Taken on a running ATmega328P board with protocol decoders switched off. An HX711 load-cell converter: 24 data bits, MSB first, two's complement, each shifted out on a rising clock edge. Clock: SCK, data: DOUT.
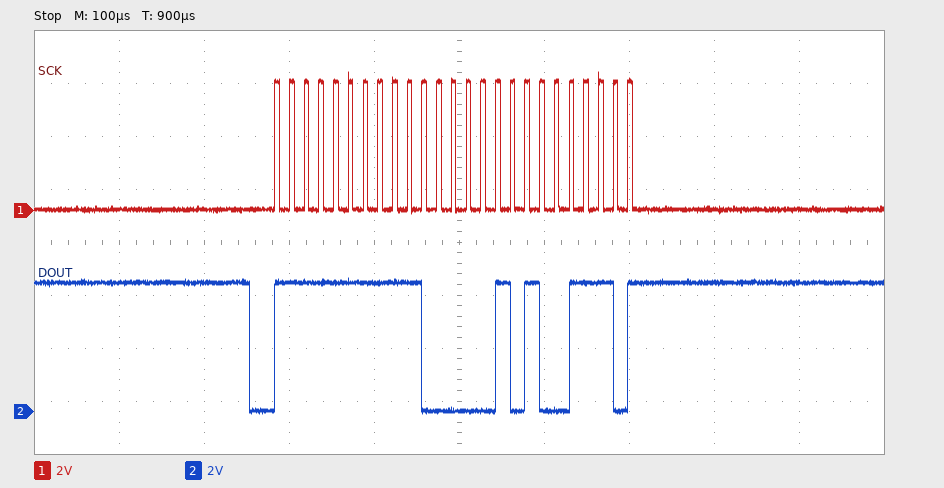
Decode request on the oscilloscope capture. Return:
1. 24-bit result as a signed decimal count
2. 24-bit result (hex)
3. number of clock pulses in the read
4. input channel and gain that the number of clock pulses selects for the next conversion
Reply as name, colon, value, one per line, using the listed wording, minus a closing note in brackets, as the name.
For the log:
24-bit result as a signed decimal count: -16050
24-bit result: 0xFFC14E
number of clock pulses in the read: 25
input channel and gain that the number of clock pulses selects for the next conversion: channel A, gain 128
